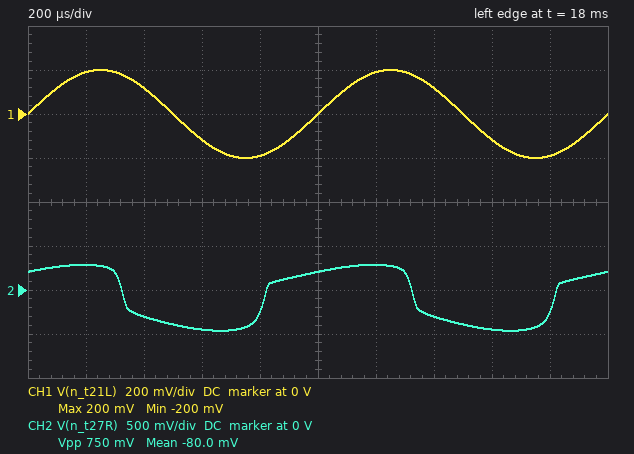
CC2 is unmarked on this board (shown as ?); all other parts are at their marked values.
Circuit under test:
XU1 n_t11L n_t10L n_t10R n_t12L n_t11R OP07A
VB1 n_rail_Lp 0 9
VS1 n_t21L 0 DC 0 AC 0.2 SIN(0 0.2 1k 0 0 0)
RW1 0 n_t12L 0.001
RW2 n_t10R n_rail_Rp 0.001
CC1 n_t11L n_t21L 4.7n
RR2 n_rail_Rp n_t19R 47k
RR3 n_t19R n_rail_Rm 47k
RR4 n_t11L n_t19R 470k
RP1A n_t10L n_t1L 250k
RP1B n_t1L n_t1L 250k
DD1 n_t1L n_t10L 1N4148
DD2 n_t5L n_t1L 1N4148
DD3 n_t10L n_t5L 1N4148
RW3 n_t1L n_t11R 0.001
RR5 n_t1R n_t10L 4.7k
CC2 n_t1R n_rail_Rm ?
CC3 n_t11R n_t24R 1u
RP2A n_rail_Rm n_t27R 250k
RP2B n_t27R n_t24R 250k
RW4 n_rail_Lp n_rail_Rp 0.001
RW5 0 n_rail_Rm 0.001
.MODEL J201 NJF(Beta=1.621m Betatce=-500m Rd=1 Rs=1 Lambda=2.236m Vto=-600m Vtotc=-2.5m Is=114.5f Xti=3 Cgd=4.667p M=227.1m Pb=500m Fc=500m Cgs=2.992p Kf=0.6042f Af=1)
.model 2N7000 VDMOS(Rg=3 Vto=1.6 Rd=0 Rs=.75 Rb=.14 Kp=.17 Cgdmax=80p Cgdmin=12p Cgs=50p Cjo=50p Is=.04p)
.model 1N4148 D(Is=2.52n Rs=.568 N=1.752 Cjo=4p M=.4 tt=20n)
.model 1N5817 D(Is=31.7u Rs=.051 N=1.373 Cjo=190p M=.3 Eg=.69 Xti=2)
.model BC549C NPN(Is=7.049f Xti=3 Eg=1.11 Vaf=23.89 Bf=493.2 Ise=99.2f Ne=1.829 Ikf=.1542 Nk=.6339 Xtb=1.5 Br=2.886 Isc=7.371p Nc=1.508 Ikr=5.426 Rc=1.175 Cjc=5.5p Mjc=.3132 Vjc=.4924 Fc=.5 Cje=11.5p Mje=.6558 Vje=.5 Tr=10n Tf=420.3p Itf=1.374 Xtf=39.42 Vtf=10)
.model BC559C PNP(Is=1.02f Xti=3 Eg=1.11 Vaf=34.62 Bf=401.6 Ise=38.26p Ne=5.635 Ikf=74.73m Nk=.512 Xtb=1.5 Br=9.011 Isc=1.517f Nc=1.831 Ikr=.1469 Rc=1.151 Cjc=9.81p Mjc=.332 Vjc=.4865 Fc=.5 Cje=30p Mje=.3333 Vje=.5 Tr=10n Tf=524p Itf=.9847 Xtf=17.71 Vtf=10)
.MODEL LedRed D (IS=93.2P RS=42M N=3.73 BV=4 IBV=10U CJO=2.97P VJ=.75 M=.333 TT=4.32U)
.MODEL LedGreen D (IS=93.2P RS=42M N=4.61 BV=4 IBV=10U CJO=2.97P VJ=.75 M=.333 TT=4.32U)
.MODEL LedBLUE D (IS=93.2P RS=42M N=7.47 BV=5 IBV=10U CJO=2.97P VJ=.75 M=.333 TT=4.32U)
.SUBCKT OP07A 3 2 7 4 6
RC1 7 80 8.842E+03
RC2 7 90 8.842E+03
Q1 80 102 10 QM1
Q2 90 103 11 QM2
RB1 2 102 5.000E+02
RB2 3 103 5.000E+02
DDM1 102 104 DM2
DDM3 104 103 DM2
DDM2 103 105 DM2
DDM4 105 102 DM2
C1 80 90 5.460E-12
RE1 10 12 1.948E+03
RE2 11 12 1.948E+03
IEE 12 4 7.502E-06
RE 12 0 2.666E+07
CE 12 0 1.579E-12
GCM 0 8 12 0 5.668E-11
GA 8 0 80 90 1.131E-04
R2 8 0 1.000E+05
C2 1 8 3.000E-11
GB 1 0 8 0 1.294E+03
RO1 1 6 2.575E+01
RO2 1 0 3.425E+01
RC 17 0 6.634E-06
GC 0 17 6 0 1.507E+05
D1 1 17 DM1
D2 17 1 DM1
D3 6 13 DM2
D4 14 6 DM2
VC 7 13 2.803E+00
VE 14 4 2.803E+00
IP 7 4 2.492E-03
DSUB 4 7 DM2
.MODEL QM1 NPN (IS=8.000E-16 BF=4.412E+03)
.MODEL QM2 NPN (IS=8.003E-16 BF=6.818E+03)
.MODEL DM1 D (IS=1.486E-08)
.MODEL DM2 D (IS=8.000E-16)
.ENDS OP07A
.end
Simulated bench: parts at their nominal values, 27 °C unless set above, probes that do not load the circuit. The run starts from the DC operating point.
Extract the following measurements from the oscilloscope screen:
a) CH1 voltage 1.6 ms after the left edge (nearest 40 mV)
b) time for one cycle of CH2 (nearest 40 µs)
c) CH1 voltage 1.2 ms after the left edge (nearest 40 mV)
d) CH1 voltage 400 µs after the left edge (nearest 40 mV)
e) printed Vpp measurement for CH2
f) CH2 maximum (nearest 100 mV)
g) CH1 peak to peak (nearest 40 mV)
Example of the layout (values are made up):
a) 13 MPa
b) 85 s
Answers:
a) -120 mV
b) 1.00 ms
c) 200 mV
d) 120 mV
e) 750 mV
f) 300 mV
g) 400 mV
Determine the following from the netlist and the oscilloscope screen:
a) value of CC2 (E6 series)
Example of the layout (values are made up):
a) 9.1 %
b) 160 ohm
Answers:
a) 15 nF
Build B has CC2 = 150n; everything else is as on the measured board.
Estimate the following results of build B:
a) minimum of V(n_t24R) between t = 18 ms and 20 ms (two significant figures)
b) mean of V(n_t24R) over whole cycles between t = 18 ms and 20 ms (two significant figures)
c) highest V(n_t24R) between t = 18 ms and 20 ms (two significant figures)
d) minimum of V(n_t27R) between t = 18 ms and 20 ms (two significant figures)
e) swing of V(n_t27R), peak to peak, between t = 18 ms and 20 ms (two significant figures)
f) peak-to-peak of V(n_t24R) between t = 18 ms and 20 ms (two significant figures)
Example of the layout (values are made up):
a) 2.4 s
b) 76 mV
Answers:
a) -1.1 V
b) -190 mV
c) 640 mV
d) -530 mV
e) 850 mV
f) 1.7 V
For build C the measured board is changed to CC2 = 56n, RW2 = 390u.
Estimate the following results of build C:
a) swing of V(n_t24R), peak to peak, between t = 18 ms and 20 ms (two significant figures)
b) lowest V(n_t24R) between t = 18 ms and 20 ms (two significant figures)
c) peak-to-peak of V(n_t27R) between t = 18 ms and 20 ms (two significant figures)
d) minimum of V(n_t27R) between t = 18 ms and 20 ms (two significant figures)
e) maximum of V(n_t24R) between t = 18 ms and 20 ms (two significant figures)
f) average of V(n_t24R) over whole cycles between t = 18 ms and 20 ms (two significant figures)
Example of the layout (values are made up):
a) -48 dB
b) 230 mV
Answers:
a) 1.7 V
b) -1.0 V
c) 840 mV
d) -520 mV
e) 630 mV
f) -180 mV
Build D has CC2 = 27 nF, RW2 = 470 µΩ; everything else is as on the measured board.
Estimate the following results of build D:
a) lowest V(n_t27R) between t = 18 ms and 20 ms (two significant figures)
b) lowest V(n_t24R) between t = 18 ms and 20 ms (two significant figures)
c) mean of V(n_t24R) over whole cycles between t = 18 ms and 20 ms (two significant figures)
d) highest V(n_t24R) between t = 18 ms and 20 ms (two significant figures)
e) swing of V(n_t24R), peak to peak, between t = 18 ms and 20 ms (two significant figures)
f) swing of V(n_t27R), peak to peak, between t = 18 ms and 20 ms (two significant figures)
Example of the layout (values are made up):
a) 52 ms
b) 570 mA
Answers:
a) -500 mV
b) -990 mV
c) -170 mV
d) 610 mV
e) 1.6 V
f) 800 mV
